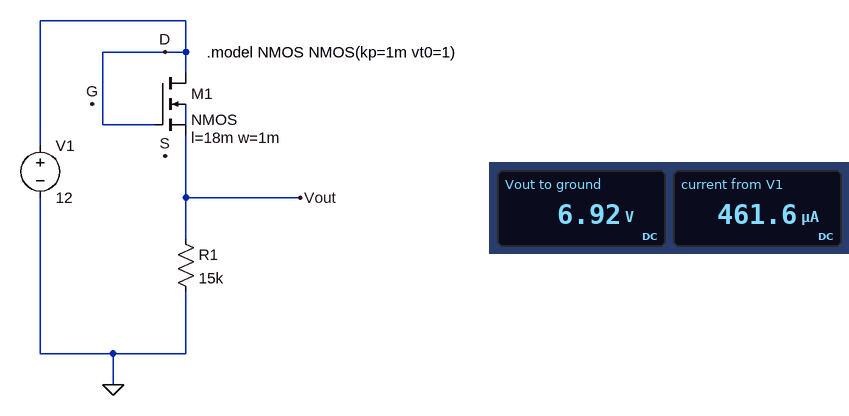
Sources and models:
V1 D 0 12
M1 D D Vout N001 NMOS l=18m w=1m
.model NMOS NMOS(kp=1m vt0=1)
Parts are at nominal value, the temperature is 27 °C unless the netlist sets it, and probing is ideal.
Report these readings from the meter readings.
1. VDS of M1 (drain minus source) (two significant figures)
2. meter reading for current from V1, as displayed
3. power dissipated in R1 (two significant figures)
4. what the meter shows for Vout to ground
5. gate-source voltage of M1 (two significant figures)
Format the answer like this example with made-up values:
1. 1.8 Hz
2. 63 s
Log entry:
1. 5.1 V
2. 461.6 µA
3. 3.2 mW
4. 6.92 V
5. 5.1 V
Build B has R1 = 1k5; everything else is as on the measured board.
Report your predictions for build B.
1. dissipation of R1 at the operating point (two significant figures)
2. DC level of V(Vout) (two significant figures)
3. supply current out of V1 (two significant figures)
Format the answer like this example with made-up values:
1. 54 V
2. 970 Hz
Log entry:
1. 5.2 mW
2. 2.8 V
3. 1.9 mA
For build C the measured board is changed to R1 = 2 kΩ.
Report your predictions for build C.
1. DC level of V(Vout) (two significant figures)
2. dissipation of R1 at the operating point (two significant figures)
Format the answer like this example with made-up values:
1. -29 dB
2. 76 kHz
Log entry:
1. 3.3 V
2. 5.4 mW
